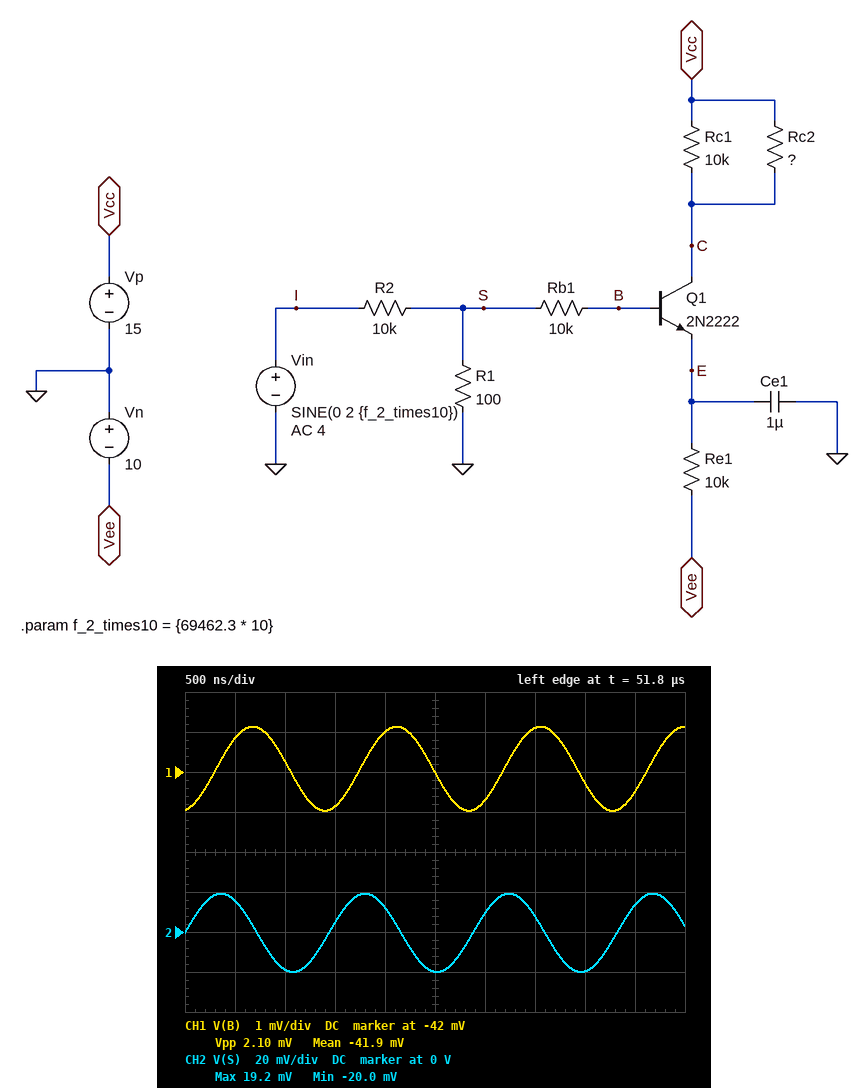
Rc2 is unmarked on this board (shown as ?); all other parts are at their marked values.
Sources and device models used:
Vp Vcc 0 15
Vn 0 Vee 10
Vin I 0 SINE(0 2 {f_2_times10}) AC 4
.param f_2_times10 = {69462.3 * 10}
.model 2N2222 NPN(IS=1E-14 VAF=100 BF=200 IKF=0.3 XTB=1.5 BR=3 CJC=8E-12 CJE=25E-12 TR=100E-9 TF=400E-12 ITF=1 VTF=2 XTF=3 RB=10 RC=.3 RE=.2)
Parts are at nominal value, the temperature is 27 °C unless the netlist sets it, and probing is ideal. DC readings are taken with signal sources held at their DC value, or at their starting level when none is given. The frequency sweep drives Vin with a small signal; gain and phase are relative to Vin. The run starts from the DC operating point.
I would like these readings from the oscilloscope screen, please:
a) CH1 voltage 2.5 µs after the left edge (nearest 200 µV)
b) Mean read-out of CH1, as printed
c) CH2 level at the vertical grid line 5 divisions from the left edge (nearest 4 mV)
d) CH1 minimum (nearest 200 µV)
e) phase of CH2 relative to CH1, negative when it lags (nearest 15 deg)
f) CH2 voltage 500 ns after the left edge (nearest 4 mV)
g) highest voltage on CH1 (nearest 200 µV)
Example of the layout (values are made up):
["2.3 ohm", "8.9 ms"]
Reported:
["-42.0 mV", "-41.9 mV", "-20 mV", "-43.0 mV", "75 deg", "16 mV", "-40.8 mV"]
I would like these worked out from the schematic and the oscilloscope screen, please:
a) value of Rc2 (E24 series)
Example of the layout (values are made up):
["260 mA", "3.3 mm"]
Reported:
["5.1 kΩ"]
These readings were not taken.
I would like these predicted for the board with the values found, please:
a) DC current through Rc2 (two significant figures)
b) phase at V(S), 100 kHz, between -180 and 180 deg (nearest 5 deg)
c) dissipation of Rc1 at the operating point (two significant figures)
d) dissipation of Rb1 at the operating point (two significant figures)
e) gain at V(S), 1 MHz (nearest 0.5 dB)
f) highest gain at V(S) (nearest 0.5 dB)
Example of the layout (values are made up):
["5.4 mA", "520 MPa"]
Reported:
["610 µA", "0 deg", "980 µW", "170 nW", "-40.0 dB", "-40.0 dB"]
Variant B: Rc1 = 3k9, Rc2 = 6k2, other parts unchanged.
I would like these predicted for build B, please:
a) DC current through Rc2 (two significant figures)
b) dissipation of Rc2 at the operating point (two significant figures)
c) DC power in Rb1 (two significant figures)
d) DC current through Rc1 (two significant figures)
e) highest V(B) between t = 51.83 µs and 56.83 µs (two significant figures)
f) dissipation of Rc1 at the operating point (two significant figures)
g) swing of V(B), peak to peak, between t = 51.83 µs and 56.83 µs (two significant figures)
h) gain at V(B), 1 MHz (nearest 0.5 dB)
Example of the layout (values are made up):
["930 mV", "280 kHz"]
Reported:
["360 µA", "790 µW", "170 nW", "570 µA", "-40 mV", "1.3 mW", "2.8 mV", "-66.0 dB"]
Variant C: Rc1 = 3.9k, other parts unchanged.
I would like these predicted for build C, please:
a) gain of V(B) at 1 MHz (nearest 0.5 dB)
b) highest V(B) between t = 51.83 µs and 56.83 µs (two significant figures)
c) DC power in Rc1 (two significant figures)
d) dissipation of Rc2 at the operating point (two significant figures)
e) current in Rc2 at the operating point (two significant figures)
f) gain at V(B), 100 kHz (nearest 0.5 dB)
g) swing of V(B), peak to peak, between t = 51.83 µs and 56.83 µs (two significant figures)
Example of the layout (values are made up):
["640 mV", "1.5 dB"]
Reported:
["-65.5 dB", "-40 mV", "1.1 mW", "820 µW", "400 µA", "-50.0 dB", "3.0 mV"]
